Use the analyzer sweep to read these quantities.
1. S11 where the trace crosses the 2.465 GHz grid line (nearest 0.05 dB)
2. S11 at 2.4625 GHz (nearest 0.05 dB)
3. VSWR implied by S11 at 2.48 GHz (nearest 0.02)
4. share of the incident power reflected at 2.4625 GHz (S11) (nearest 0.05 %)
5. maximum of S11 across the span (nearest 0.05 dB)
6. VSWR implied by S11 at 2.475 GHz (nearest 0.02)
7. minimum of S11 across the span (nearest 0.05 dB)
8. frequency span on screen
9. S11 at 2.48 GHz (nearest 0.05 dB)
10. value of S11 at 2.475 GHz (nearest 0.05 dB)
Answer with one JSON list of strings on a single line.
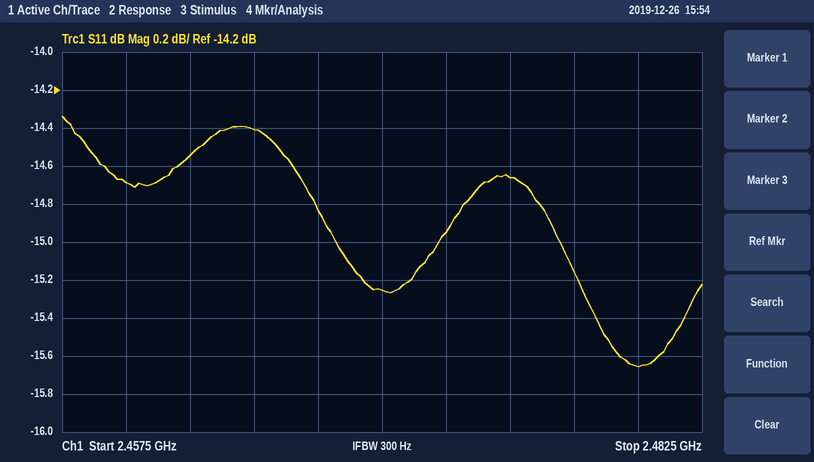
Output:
["-14.40 dB", "-14.55 dB", "1.40", "3.50 %", "-14.35 dB", "1.46", "-15.65 dB", "25 MHz", "-15.65 dB", "-14.65 dB"]
